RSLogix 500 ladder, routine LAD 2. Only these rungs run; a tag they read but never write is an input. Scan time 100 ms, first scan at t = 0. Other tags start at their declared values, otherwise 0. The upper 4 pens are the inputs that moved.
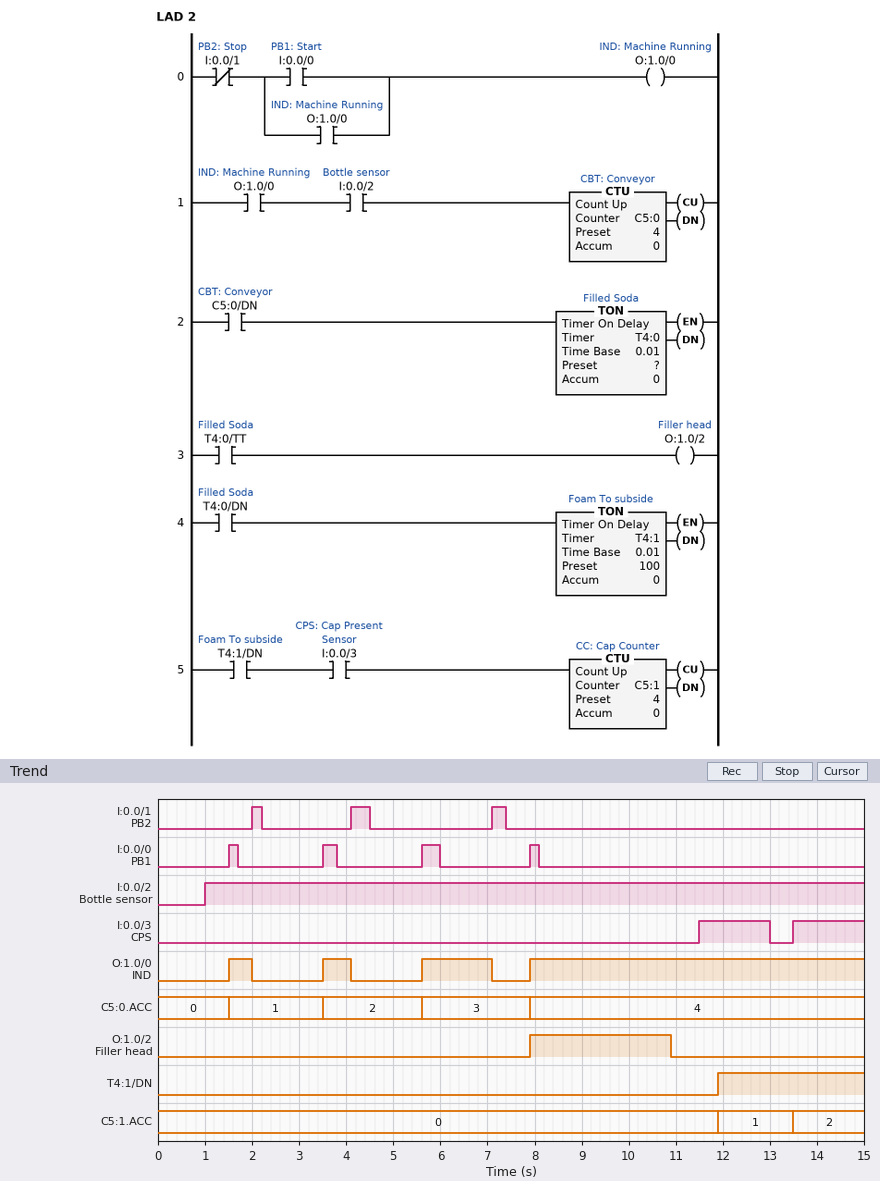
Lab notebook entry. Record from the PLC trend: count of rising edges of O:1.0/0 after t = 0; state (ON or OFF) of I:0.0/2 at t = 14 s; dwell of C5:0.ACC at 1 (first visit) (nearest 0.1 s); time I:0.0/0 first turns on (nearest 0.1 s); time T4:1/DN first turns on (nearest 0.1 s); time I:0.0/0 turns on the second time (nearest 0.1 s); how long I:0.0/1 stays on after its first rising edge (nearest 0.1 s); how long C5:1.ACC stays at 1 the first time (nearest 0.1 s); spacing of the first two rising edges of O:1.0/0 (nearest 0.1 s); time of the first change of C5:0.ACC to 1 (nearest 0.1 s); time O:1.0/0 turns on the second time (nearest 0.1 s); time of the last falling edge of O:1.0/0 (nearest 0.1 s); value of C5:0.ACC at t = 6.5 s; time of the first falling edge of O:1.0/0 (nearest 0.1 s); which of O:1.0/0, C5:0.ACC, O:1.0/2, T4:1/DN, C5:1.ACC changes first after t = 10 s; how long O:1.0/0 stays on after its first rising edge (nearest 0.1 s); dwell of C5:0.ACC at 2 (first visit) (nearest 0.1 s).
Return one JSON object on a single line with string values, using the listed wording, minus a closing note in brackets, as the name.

{"count of rising edges of O:1.0/0 after t = 0": "4", "state (ON or OFF) of I:0.0/2 at t = 14 s": "ON", "dwell of C5:0.ACC at 1 (first visit)": "2.0 s", "time I:0.0/0 first turns on": "1.5 s", "time T4:1/DN first turns on": "11.9 s", "time I:0.0/0 turns on the second time": "3.5 s", "how long I:0.0/1 stays on after its first rising edge": "0.2 s", "how long C5:1.ACC stays at 1 the first time": "1.6 s", "spacing of the first two rising edges of O:1.0/0": "2.0 s", "time of the first change of C5:0.ACC to 1": "1.5 s", "time O:1.0/0 turns on the second time": "3.5 s", "time of the last falling edge of O:1.0/0": "7.1 s", "value of C5:0.ACC at t = 6.5 s": "3", "time of the first falling edge of O:1.0/0": "2.0 s", "which of O:1.0/0, C5:0.ACC, O:1.0/2, T4:1/DN, C5:1.ACC changes first after t = 10 s": "O:1.0/2", "how long O:1.0/0 stays on after its first rising edge": "0.5 s", "dwell of C5:0.ACC at 2 (first visit)": "2.1 s"}
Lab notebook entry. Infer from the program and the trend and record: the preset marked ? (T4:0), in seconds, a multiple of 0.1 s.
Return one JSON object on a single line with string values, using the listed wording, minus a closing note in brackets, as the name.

{"the preset marked ? (T4:0), in seconds, a multiple of 0.1 s": "3.0 s"}
